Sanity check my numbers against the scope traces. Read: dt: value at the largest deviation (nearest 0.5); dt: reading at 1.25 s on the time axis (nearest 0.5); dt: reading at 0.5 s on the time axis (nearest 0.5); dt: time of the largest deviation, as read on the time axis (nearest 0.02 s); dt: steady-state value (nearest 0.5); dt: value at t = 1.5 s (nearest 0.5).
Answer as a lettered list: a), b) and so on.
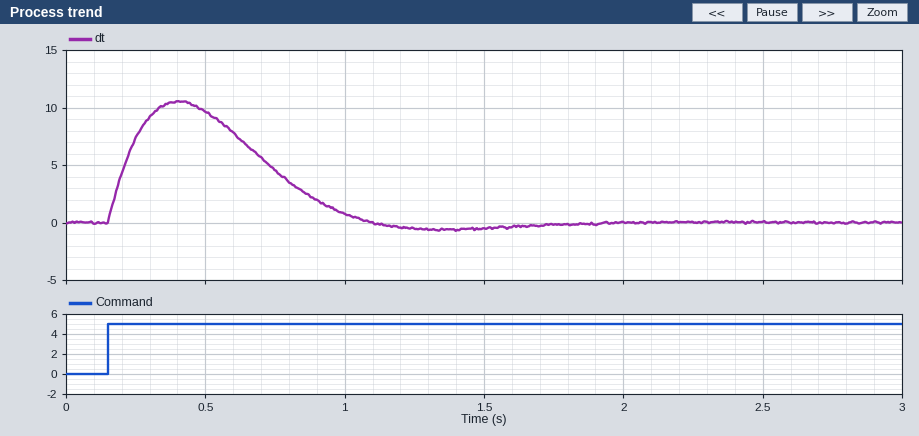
a) 10.5
b) -0.5
c) 9.5
d) 0.40 s
e) 0.0
f) -0.5
